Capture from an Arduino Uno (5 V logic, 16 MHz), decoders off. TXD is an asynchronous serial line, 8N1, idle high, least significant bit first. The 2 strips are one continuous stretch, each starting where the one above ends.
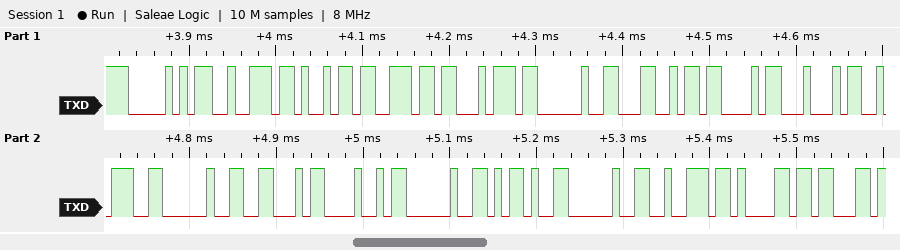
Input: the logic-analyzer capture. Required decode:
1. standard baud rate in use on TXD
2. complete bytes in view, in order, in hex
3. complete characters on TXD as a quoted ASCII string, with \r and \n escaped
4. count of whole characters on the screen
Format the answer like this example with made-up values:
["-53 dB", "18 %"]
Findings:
["115200 baud", "50 72 69 6E 74 20 4C 43 44 3A 20 46 48 20 2D 20 72 61 63", "\"Print LCD: FH - rac\"", "19"]
